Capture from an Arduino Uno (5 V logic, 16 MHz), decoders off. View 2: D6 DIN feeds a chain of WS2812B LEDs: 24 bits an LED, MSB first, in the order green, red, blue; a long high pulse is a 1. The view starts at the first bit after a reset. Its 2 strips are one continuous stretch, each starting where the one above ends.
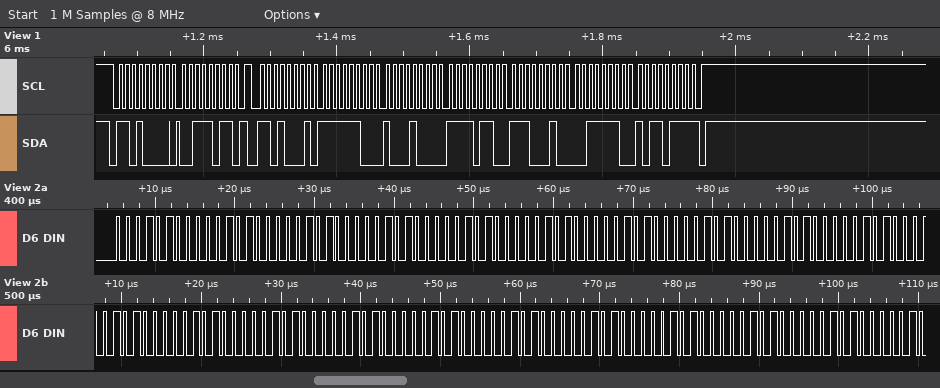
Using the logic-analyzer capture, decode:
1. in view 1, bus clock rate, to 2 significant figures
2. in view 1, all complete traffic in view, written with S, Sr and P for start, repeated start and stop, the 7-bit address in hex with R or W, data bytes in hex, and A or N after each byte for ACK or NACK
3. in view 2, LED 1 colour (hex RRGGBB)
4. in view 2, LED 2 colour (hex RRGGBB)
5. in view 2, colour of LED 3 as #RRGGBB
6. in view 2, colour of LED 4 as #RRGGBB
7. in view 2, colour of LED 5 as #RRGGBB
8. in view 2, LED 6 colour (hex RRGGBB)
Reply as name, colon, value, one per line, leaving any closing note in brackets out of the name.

in view 1, bus clock rate, to 2 significant figures: 100 kHz
in view 1, all complete traffic in view, written with S, Sr and P for start, repeated start and stop, the 7-bit address in hex with R or W, data bytes in hex, and A or N after each byte for ACK or NACK: S 68W A 3B A Sr 68R A FC A 88 A F6 A E2 A 3E A B7 N P
in view 2, LED 1 colour: #141414
in view 2, LED 2 colour: #141414
in view 2, colour of LED 3 as #RRGGBB: #141414
in view 2, colour of LED 4 as #RRGGBB: #141414
in view 2, colour of LED 5 as #RRGGBB: #141414
in view 2, LED 6 colour: #141414
